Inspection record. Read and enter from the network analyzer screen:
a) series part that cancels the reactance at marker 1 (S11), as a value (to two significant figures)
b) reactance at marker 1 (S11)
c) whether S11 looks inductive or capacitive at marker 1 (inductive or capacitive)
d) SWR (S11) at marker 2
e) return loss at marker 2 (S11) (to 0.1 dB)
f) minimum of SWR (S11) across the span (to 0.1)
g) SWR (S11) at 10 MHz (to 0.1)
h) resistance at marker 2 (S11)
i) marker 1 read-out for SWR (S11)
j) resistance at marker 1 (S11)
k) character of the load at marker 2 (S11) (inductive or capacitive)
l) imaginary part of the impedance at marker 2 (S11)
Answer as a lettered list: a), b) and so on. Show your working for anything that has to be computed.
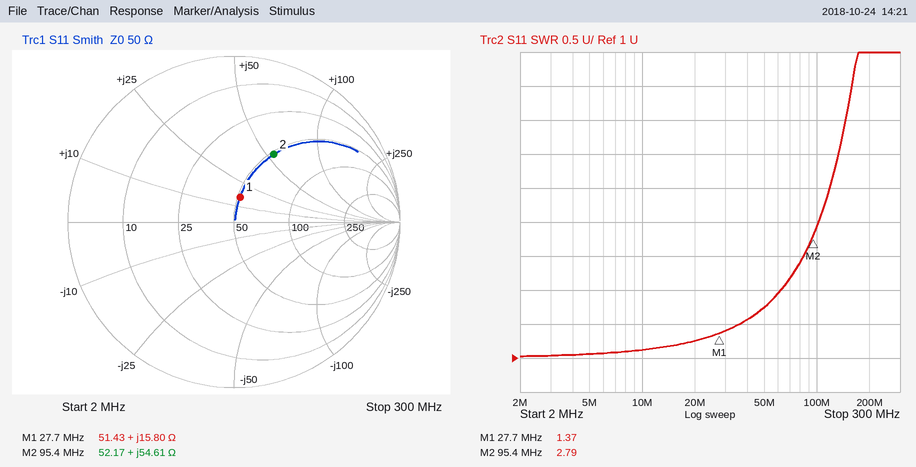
a) C = 1/(2π × 27.7 MHz × 15.8 Ω) ≈ 364 pF, so 360 pF to two significant figures
b) +15.80 Ω
c) inductive
d) 2.79
e) 6.5 dB
f) 1.0
g) 1.1
h) 52.17 Ω
i) 1.37
j) 51.43 Ω
k) inductive
l) +54.61 Ω
